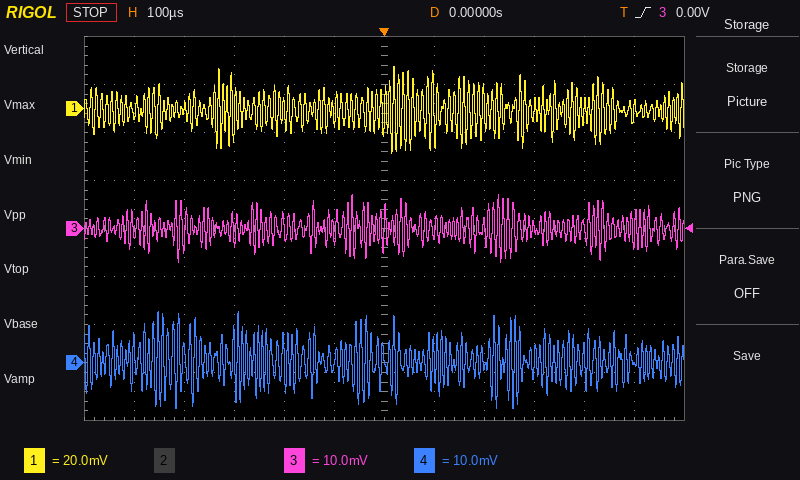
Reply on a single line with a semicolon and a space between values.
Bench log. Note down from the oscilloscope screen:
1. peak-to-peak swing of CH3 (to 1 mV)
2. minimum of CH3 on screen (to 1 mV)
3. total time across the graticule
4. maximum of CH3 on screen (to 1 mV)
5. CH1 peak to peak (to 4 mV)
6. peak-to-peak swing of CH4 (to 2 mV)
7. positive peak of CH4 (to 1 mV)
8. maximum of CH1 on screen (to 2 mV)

14 mV; -7 mV; 1.2 ms; 7 mV; 36 mV; 20 mV; 11 mV; 18 mV
